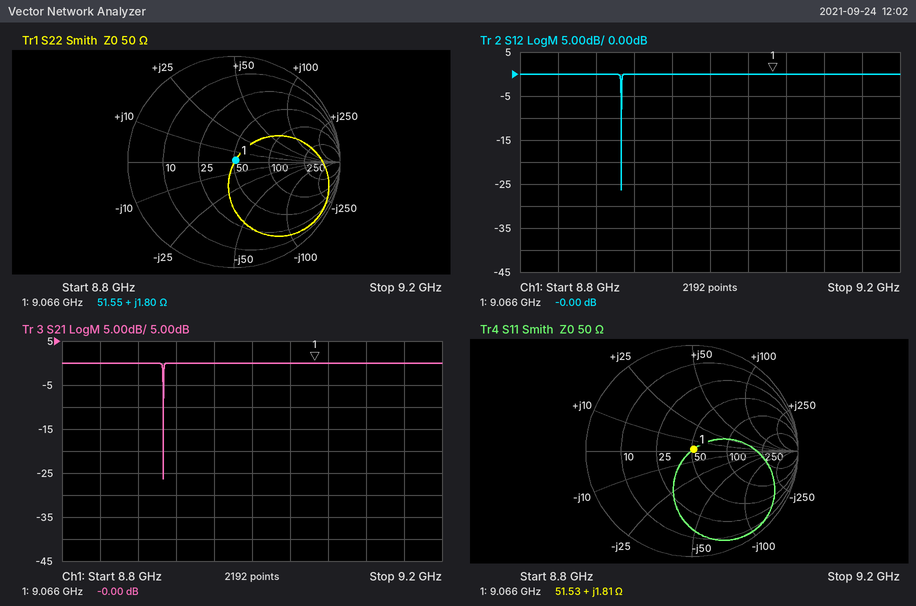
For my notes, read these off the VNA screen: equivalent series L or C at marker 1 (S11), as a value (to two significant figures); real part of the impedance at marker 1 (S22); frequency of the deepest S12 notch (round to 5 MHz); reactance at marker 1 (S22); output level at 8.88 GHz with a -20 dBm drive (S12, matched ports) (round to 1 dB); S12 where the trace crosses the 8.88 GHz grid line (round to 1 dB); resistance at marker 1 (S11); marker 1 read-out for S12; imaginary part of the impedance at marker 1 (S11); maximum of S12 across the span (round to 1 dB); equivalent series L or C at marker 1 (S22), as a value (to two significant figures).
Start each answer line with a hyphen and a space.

- 32 pH
- 51.55 Ω
- 8.905 GHz
- +1.80 Ω
- -20 dBm
- 0 dB
- 51.53 Ω
- -0.00 dB
- +1.81 Ω
- 0 dB
- 32 pH
